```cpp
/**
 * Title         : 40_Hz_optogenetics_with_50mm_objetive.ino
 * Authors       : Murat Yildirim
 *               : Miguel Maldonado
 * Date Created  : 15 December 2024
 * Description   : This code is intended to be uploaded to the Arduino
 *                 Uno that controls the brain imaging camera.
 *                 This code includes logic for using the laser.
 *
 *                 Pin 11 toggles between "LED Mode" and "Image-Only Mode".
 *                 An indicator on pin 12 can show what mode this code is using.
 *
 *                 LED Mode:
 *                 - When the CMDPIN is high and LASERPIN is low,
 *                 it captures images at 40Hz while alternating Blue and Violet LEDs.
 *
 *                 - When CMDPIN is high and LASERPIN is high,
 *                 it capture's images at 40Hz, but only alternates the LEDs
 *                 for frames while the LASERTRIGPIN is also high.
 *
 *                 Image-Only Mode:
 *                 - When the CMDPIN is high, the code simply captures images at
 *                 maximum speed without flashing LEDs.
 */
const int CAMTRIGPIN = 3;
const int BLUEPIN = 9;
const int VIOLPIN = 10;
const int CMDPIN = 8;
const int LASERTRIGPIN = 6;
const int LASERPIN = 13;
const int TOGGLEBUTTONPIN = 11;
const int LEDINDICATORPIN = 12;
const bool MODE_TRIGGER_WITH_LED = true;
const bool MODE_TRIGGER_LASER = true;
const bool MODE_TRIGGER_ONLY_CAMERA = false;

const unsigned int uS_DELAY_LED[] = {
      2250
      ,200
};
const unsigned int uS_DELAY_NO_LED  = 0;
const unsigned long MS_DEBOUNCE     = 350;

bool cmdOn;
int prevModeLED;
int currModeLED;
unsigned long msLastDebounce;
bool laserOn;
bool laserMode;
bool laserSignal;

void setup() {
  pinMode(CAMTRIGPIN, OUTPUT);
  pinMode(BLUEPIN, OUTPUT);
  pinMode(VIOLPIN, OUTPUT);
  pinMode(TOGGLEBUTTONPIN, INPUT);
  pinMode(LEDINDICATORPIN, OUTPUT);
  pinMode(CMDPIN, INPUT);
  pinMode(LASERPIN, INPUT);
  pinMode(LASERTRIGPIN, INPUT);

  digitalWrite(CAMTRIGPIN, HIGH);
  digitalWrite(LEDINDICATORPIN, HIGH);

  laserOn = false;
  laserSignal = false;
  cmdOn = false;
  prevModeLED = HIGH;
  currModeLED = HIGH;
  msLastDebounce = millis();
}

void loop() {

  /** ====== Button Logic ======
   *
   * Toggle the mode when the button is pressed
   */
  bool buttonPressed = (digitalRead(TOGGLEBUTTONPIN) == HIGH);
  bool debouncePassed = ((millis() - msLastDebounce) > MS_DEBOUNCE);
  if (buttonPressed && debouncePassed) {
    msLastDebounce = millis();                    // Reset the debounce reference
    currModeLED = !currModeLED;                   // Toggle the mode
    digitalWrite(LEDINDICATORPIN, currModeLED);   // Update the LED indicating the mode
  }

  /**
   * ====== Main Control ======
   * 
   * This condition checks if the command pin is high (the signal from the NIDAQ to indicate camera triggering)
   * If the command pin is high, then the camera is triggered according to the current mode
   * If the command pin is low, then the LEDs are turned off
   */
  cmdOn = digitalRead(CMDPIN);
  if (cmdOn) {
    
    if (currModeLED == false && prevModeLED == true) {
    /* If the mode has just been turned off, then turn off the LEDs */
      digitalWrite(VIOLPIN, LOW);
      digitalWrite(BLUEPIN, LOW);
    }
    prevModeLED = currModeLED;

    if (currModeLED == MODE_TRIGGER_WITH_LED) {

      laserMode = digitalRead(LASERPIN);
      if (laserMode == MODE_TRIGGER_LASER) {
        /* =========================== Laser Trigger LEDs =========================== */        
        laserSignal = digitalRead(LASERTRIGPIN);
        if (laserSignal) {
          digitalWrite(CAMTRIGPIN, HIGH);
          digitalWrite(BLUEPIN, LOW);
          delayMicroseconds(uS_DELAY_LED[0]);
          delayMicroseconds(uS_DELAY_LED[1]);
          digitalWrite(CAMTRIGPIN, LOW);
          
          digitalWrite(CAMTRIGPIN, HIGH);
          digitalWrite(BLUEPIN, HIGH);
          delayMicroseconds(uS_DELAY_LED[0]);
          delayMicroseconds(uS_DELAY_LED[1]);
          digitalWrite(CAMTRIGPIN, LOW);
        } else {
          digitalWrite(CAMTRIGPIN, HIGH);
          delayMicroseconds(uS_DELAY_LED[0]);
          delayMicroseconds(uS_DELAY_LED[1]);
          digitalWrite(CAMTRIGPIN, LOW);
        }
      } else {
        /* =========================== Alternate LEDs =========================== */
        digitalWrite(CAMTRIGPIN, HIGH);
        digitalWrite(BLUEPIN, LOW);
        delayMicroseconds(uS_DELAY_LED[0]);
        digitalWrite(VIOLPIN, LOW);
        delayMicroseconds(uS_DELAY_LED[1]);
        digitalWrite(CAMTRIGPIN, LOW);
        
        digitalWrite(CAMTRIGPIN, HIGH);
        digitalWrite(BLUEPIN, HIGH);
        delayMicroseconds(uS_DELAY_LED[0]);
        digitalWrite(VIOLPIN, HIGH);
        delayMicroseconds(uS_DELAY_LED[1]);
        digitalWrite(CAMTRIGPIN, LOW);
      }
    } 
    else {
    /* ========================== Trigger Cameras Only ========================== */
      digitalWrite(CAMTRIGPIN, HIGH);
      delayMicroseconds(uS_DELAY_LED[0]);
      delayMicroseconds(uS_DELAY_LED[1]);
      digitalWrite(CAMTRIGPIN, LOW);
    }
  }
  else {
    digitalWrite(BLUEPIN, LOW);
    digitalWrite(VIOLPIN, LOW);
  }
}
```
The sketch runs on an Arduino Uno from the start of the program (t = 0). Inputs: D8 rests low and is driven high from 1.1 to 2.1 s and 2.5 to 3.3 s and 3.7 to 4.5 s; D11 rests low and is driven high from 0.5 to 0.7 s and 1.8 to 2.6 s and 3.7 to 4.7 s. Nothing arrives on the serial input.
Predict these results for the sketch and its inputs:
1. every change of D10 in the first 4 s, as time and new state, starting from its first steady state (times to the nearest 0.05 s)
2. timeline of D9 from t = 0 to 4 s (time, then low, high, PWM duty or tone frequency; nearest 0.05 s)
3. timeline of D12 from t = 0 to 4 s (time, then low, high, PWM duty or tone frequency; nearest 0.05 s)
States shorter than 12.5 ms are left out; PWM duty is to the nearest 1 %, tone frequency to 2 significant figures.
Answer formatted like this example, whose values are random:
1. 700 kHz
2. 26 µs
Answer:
1. 0 s low; 1.8 s tone 200 Hz; 2.1 s low; 2.5 s tone 200 Hz; 3.3 s low
2. 0 s low; 1.8 s tone 200 Hz; 2.1 s low; 2.5 s tone 200 Hz; 3.3 s low
3. 0 s high; 0.5 s low; 1.8 s high; 2.15 s low; 2.5 s high; 3.7 s low
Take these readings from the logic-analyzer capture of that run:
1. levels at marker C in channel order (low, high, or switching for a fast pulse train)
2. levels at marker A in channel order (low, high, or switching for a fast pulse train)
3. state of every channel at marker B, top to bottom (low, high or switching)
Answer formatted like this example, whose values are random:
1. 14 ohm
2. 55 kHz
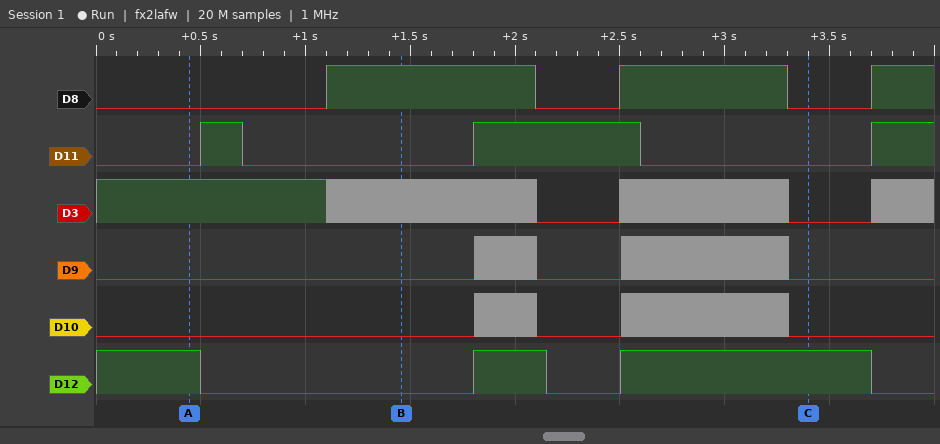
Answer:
1. D8 low, D11 low, D3 low, D9 low, D10 low, D12 high
2. D8 low, D11 low, D3 high, D9 low, D10 low, D12 high
3. D8 high, D11 low, D3 switching, D9 low, D10 low, D12 low
